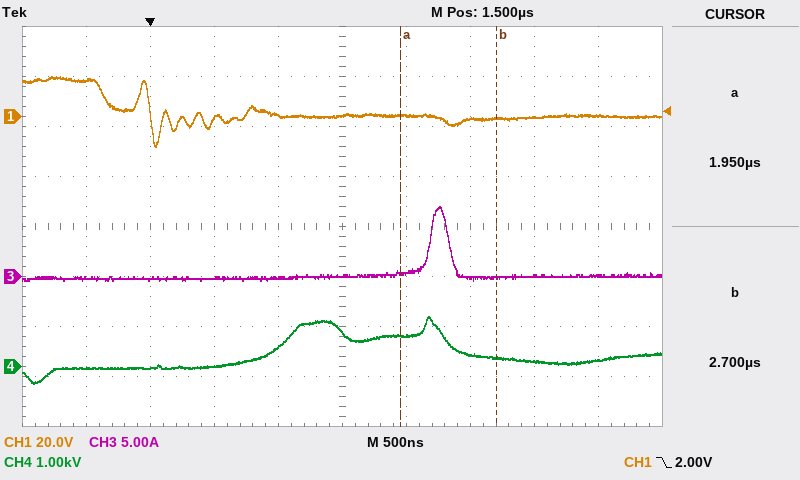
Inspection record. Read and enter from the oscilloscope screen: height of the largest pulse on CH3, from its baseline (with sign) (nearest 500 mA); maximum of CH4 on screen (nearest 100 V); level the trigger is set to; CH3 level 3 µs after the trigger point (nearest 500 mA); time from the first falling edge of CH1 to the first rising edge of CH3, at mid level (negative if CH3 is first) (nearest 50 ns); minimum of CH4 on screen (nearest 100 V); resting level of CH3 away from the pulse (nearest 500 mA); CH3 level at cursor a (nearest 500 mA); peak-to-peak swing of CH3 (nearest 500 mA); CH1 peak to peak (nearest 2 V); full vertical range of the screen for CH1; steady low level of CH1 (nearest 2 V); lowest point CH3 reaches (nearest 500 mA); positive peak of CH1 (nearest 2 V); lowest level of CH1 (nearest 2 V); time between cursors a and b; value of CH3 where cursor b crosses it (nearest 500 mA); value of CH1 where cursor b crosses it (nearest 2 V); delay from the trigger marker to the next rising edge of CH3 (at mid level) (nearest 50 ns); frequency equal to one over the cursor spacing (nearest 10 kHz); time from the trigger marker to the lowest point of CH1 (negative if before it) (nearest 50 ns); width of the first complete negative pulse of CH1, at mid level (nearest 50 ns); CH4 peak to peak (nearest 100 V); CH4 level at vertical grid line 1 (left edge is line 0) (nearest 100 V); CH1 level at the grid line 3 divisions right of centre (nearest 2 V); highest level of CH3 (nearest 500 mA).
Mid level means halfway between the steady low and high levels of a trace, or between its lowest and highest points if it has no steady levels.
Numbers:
+7.0 A
1.0 kV
2.00 V
0.0 A
+2.55 µs
-300 V
0.0 A
500 mA
7.5 A
28 V
160 V
0 V
-500 mA
16 V
-12 V
750 ns
0.0 A
0 V
2.20 µs
1.33 MHz
+50 ns
250 ns
1.3 kV
0.0 kV
0 V
7.0 A
